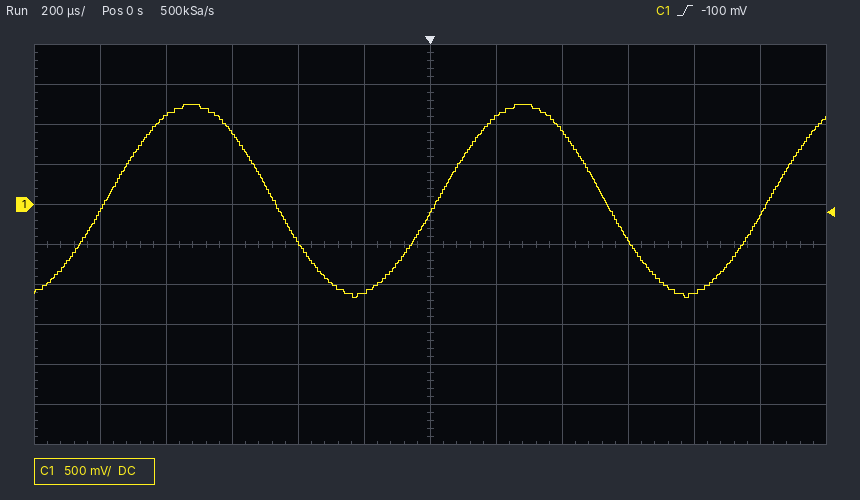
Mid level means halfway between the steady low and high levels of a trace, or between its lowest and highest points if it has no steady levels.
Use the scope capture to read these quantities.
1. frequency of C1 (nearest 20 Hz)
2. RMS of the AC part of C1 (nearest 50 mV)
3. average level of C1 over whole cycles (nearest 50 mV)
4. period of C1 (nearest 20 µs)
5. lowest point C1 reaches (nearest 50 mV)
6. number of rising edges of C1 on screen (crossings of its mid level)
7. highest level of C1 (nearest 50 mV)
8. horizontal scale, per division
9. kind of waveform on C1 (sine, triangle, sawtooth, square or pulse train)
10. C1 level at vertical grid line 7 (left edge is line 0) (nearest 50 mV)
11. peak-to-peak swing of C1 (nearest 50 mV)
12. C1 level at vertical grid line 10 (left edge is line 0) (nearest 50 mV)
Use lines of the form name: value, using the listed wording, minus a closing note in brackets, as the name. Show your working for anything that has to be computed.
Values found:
frequency of C1: 1 / 1.00 ms ≈ 1.00 kHz
RMS of the AC part of C1: 2.40 V / (2√2) ≈ 849 mV, so 850 mV to the nearest 50 mV
average level of C1 over whole cycles: (1.25 V + (-1.15 V)) / 2 ≈ 50 mV
period of C1: 1.00 ms
lowest point C1 reaches: -1.15 V
number of rising edges of C1 on screen: 3
highest level of C1: 1.25 V
horizontal scale, per division: 200 µs
kind of waveform on C1: sine
C1 level at vertical grid line 7 (left edge is line 0): 1.10 V
peak-to-peak swing of C1: 1.25 V − (-1.15 V) = 2.40 V
C1 level at vertical grid line 10 (left edge is line 0): -1.10 V
